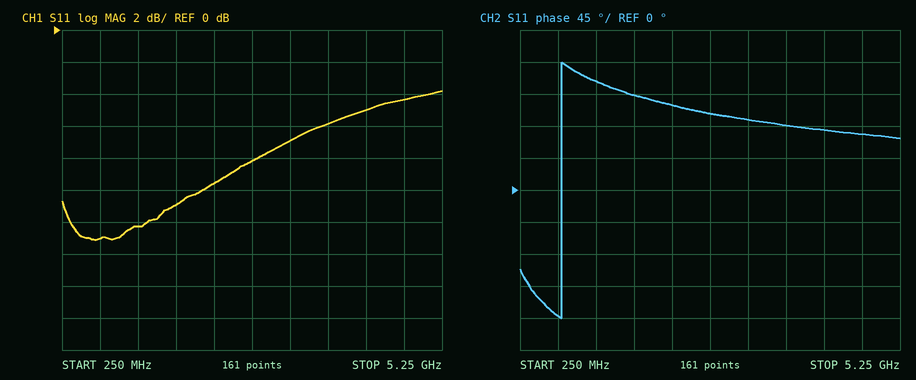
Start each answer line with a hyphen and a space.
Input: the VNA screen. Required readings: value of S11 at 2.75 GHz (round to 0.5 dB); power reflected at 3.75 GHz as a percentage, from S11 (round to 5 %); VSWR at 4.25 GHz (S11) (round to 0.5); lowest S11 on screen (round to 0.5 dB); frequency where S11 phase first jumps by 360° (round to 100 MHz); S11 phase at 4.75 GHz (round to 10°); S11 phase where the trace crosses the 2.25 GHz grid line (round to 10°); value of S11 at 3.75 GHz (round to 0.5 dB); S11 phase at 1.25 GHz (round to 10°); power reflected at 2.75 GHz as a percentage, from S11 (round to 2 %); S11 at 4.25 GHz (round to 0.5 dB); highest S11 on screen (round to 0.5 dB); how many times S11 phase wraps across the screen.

- -8.0 dB
- 25 %
- 3.5
- -13.0 dB
- 800 MHz
- 80°
- 120°
- -6.0 dB
- 150°
- 16 %
- -5.0 dB
- -4.0 dB
- 1
